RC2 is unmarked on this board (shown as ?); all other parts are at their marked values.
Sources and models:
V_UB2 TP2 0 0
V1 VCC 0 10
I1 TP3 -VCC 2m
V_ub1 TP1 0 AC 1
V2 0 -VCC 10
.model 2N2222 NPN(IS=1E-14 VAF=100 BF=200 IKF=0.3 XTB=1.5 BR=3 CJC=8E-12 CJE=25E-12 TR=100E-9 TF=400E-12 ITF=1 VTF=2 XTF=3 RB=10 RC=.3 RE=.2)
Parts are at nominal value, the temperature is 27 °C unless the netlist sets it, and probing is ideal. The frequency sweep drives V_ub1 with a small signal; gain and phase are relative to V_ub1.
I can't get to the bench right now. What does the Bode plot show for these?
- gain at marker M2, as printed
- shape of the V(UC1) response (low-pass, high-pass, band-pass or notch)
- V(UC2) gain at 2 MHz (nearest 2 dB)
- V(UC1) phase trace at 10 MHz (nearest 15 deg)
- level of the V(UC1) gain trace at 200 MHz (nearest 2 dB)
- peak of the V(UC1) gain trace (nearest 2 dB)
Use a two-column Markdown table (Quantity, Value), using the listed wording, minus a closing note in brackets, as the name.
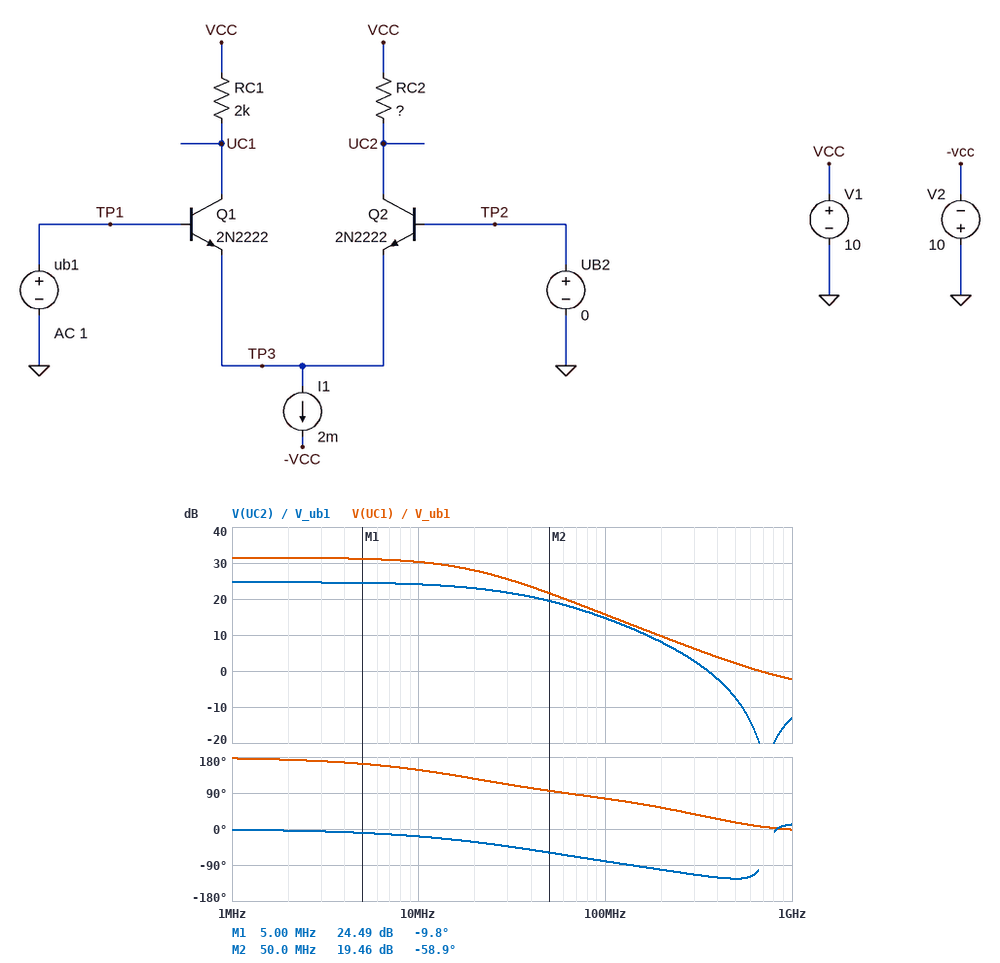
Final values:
| Quantity | Value |
|---|---|
| gain at marker M2, as printed | 19.46 dB |
| shape of the V(UC1) response | low-pass |
| V(UC2) gain at 2 MHz | 24 dB |
| V(UC1) phase trace at 10 MHz | 150 deg |
| level of the V(UC1) gain trace at 200 MHz | 10 dB |
| peak of the V(UC1) gain trace | 32 dB |
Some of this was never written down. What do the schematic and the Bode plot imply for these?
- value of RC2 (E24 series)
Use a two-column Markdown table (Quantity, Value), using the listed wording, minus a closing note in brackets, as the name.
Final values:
| Quantity | Value |
|---|---|
| value of RC2 | 910 Ω |
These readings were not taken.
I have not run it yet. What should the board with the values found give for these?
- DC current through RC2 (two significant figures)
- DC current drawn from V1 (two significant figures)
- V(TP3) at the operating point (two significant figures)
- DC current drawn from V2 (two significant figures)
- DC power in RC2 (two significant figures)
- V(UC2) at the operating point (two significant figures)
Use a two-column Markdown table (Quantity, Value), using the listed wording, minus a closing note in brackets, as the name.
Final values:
| Quantity | Value |
|---|---|
| DC current through RC2 | 1.0 mA |
| DC current drawn from V1 | 2.0 mA |
| V(TP3) at the operating point | -650 mV |
| DC current drawn from V2 | 2.0 mA |
| DC power in RC2 | 910 µW |
| V(UC2) at the operating point | 9.1 V |
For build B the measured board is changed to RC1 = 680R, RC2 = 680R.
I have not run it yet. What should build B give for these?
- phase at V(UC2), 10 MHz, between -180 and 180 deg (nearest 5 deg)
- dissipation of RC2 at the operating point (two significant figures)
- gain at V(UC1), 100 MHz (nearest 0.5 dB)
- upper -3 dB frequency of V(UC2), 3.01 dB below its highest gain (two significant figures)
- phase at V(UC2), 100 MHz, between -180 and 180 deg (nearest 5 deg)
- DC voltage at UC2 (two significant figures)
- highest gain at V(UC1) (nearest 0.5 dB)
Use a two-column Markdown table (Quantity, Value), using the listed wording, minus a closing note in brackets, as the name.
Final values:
| Quantity | Value |
|---|---|
| phase at V(UC2), 10 MHz, between -180 and 180 deg | -15 deg |
| dissipation of RC2 at the operating point | 670 µW |
| gain at V(UC1), 100 MHz | 15.0 dB |
| upper -3 dB frequency of V(UC2), 3.01 dB below its highest gain | 46 MHz |
| phase at V(UC2), 100 MHz, between -180 and 180 deg | -75 deg |
| DC voltage at UC2 | 9.3 V |
| highest gain at V(UC1) | 22.0 dB |
